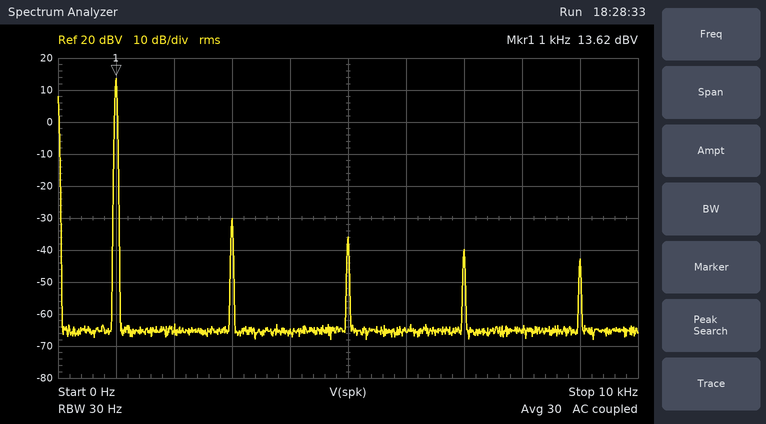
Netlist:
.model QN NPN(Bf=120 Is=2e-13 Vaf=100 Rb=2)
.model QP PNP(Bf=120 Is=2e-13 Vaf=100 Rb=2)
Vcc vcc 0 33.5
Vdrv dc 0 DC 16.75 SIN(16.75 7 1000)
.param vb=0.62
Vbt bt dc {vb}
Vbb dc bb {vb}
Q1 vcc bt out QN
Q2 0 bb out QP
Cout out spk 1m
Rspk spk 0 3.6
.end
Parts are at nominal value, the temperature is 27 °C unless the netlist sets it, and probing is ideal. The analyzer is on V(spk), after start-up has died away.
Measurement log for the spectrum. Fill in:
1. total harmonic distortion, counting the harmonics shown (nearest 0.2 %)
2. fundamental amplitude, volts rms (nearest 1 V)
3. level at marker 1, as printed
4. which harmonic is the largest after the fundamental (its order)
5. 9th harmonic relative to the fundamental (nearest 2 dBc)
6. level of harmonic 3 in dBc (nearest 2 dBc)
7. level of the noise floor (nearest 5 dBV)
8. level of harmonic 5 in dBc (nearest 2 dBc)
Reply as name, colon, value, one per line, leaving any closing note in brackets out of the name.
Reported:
total harmonic distortion, counting the harmonics shown: 0.8 %
fundamental amplitude, volts rms: 5 V
level at marker 1, as printed: 13.62 dBV
which harmonic is the largest after the fundamental: 3
9th harmonic relative to the fundamental: -56 dBc
level of harmonic 3 in dBc: -44 dBc
level of the noise floor: -65 dBV
level of harmonic 5 in dBc: -50 dBc
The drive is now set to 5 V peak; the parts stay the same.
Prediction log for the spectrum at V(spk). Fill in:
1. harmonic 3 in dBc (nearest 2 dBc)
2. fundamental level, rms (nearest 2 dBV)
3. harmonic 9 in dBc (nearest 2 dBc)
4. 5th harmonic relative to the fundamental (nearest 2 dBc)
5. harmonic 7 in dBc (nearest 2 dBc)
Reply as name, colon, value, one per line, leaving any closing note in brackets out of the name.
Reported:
harmonic 3 in dBc: -42 dBc
fundamental level, rms: 10 dBV
harmonic 9 in dBc: -54 dBc
5th harmonic relative to the fundamental: -48 dBc
harmonic 7 in dBc: -52 dBc
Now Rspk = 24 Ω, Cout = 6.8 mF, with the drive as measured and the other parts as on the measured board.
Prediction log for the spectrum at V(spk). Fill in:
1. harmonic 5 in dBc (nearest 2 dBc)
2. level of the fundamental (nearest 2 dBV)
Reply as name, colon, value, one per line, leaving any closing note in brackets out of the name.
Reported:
harmonic 5 in dBc: -56 dBc
level of the fundamental: 14 dBV
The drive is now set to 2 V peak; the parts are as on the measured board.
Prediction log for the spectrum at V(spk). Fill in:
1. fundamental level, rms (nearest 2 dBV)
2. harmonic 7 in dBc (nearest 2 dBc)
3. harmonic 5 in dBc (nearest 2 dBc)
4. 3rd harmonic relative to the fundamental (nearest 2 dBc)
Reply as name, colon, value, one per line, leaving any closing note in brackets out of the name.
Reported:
fundamental level, rms: 2 dBV
harmonic 7 in dBc: -48 dBc
harmonic 5 in dBc: -42 dBc
3rd harmonic relative to the fundamental: -36 dBc
